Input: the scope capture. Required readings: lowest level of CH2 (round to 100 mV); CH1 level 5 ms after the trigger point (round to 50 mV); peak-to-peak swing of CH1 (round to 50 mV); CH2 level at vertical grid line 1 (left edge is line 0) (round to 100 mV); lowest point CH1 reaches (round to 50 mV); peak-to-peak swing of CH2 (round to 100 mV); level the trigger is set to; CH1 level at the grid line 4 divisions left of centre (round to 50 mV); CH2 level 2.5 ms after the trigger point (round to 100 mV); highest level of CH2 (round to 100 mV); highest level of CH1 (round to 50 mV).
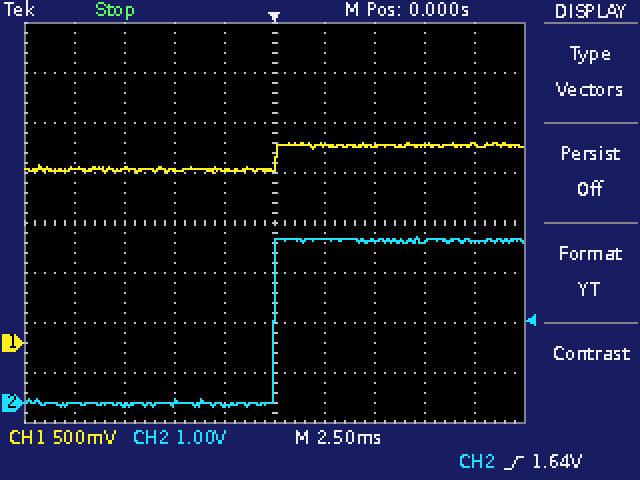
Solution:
-100 mV
1.95 V
300 mV
0.0 V
1.70 V
3.4 V
1.64 V
1.75 V
3.3 V
3.3 V
2.00 V
